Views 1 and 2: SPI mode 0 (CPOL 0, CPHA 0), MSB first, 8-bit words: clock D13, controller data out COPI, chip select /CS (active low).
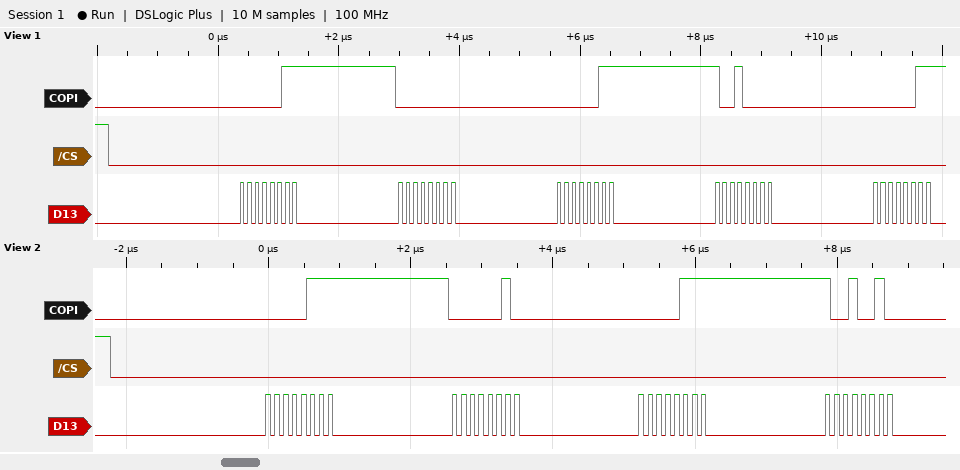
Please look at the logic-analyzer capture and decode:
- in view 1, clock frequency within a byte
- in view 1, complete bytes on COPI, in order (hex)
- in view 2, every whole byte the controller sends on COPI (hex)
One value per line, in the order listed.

8 MHz
03 00 03 90 03
07 02 07 92
